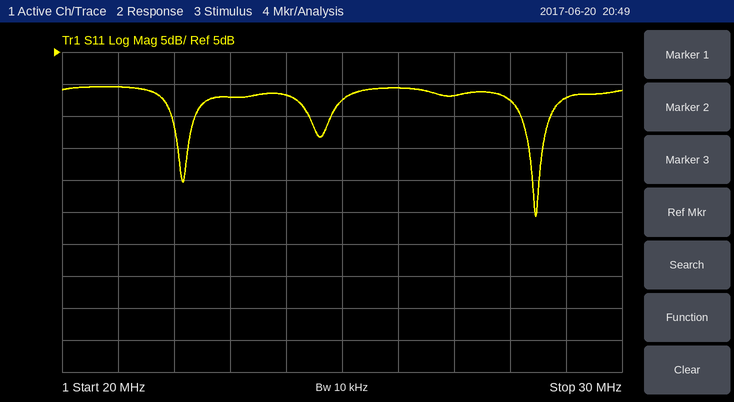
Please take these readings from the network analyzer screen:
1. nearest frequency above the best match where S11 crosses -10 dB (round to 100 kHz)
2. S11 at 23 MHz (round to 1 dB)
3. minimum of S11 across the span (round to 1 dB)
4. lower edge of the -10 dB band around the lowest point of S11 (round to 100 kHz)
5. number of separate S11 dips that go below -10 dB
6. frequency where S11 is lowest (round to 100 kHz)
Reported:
28.6 MHz
-2 dB
-21 dB
28.3 MHz
2
28.5 MHz
